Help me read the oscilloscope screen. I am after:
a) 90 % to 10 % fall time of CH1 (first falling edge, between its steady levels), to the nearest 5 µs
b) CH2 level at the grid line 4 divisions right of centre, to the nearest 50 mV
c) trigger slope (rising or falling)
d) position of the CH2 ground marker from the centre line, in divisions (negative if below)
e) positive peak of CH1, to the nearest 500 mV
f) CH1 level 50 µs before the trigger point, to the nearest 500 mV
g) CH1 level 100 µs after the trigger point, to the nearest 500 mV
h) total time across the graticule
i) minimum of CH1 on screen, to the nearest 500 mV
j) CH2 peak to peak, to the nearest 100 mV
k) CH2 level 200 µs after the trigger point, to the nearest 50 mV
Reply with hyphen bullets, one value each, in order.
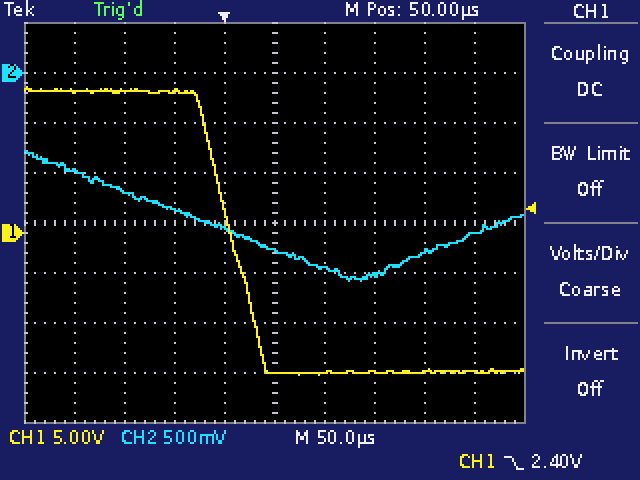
- 55 µs
- -1.60 V
- falling
- +3.0 div
- 14.5 V
- 14.0 V
- -14.0 V
- 500 µs
- -14.0 V
- 1.30 V
- -1.80 V
